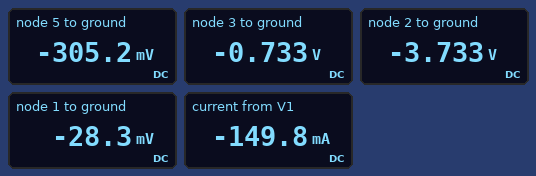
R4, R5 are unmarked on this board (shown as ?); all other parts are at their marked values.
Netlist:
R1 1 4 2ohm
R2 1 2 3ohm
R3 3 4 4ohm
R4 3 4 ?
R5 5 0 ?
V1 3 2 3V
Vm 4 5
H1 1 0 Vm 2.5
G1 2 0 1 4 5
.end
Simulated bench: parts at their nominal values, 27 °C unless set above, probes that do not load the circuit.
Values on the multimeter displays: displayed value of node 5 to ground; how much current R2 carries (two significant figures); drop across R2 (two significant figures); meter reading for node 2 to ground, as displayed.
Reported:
-305.2 mV
1.2 A
3.7 V
-3.733 V
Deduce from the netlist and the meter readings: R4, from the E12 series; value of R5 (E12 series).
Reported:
10 Ω
27 Ω
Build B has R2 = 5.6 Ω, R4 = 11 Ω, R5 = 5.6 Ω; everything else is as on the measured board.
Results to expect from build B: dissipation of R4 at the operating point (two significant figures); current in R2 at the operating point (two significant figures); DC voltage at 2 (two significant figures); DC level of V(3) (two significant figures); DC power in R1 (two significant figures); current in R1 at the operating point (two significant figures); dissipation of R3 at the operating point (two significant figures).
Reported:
12 mW
630 mA
-3.6 V
-630 mV
11 mW
75 mA
33 mW
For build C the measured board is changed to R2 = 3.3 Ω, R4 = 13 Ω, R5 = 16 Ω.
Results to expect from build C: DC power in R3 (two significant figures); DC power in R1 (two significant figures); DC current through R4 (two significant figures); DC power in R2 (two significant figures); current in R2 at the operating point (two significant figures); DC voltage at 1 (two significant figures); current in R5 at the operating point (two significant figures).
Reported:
49 mW
32 mW
34 mA
4.1 W
1.1 A
-47 mV
19 mA
